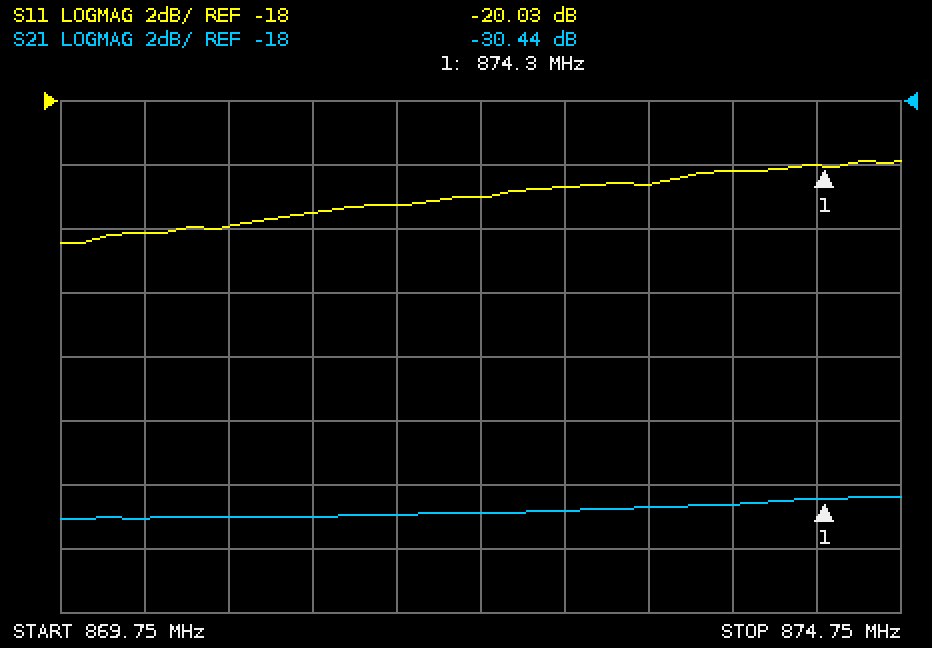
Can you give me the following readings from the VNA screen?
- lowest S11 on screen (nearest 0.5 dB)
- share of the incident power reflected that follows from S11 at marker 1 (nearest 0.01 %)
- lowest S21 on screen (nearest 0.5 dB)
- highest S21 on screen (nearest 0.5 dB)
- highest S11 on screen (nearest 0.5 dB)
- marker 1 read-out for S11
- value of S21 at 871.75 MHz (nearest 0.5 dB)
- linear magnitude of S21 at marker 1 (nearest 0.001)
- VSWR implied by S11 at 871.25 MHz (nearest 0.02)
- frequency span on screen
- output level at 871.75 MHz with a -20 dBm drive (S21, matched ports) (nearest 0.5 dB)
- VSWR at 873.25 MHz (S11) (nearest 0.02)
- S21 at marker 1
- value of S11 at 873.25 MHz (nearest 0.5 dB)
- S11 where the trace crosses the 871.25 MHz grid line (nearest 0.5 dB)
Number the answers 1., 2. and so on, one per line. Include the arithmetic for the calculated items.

1. -22.5 dB
2. 10^(-20.03/10) ≈ 0.99 %
3. -31.0 dB
4. -30.5 dB
5. -20.0 dB
6. -20.03 dB
7. -31.0 dB
8. 10^(-30.44/20) ≈ 0.030
9. |Γ| = 10^(-21.5/20) = 0.0841; VSWR = (1 + 0.0841)/(1 − 0.0841) ≈ 1.18
10. 5 MHz
11. -20 dBm + (-31.0 dB) = -51.0 dBm
12. |Γ| = 10^(-20.5/20) = 0.0944; VSWR = (1 + 0.0944)/(1 − 0.0944) ≈ 1.21, so 1.20 to the nearest 0.02
13. -30.44 dB
14. -20.5 dB
15. -21.5 dB
